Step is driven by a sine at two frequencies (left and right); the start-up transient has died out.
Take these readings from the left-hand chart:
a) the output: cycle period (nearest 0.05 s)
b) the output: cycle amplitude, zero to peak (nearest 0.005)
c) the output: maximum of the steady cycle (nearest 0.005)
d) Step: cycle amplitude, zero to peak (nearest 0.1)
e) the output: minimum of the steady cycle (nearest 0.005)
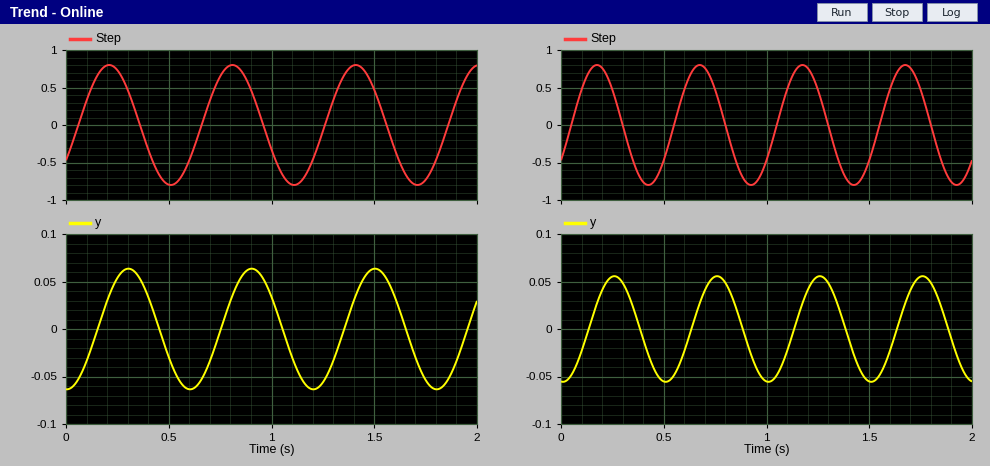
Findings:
0.60 s
0.065
0.065
0.8
-0.065
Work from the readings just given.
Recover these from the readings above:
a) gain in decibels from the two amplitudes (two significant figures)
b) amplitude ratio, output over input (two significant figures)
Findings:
-22 dB
0.081
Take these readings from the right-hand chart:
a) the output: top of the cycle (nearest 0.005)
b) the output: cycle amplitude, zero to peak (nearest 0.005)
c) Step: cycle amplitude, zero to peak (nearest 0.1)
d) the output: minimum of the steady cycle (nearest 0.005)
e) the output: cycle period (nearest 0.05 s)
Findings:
0.055
0.055
0.8
-0.055
0.50 s
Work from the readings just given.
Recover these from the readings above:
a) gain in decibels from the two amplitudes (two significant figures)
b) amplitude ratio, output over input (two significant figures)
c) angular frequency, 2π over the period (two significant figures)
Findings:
-23 dB
0.069
13 rad/s
